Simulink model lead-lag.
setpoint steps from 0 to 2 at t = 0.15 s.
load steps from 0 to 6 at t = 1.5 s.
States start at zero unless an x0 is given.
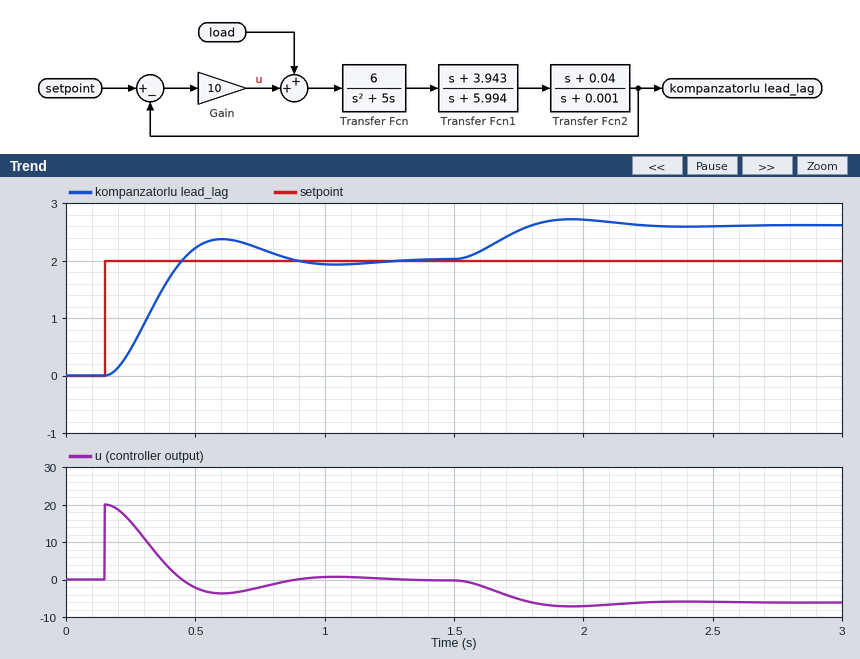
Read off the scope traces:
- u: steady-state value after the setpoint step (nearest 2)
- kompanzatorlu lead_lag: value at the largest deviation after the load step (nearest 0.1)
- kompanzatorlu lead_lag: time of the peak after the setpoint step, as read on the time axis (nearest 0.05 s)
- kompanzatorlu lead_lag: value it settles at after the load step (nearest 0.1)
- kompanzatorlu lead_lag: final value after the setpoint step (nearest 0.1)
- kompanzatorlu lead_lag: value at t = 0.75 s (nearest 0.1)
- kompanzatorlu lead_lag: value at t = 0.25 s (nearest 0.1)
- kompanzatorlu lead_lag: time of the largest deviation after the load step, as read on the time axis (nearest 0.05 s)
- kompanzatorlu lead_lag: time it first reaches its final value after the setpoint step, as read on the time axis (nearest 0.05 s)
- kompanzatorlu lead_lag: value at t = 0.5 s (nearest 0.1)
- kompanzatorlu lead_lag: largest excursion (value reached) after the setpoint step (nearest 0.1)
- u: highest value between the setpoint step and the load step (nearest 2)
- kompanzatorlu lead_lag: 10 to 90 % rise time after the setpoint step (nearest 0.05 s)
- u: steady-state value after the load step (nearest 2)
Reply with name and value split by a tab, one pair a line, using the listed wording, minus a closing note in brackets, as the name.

u: steady-state value after the setpoint step	0
kompanzatorlu lead_lag: value at the largest deviation after the load step	2.7
kompanzatorlu lead_lag: time of the peak after the setpoint step, as read on the time axis	0.60 s
kompanzatorlu lead_lag: value it settles at after the load step	2.6
kompanzatorlu lead_lag: final value after the setpoint step	2.0
kompanzatorlu lead_lag: value at t = 0.75 s	2.2
kompanzatorlu lead_lag: value at t = 0.25 s	0.5
kompanzatorlu lead_lag: time of the largest deviation after the load step, as read on the time axis	1.95 s
kompanzatorlu lead_lag: time it first reaches its final value after the setpoint step, as read on the time axis	0.45 s
kompanzatorlu lead_lag: value at t = 0.5 s	2.2
kompanzatorlu lead_lag: largest excursion (value reached) after the setpoint step	2.4
u: highest value between the setpoint step and the load step	20
kompanzatorlu lead_lag: 10 to 90 % rise time after the setpoint step	0.20 s
u: steady-state value after the load step	-6
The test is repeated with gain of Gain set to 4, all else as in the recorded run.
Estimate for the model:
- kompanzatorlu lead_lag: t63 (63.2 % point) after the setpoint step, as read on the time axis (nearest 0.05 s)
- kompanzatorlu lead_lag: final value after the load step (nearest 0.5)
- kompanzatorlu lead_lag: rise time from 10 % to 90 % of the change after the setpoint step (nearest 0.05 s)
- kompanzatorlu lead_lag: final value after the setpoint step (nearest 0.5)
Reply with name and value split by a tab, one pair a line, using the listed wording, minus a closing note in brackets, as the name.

kompanzatorlu lead_lag: t63 (63.2 % point) after the setpoint step, as read on the time axis	0.50 s
kompanzatorlu lead_lag: final value after the load step	3.5
kompanzatorlu lead_lag: rise time from 10 % to 90 % of the change after the setpoint step	0.45 s
kompanzatorlu lead_lag: final value after the setpoint step	2.0
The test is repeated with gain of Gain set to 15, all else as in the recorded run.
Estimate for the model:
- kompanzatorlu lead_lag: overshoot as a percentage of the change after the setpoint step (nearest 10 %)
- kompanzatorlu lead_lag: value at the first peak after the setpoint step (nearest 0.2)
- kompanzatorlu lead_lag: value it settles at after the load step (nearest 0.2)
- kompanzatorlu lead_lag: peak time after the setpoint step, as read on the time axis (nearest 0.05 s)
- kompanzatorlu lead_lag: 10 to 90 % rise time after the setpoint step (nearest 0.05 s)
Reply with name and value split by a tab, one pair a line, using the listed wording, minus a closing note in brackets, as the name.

kompanzatorlu lead_lag: overshoot as a percentage of the change after the setpoint step	30 %
kompanzatorlu lead_lag: value at the first peak after the setpoint step	2.6
kompanzatorlu lead_lag: value it settles at after the load step	2.4
kompanzatorlu lead_lag: peak time after the setpoint step, as read on the time axis	0.50 s
kompanzatorlu lead_lag: 10 to 90 % rise time after the setpoint step	0.15 s
